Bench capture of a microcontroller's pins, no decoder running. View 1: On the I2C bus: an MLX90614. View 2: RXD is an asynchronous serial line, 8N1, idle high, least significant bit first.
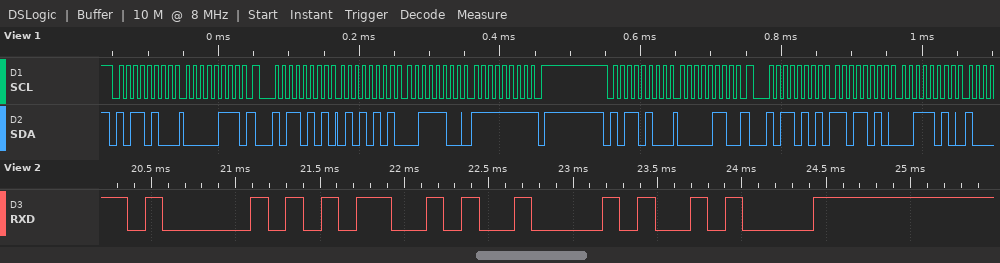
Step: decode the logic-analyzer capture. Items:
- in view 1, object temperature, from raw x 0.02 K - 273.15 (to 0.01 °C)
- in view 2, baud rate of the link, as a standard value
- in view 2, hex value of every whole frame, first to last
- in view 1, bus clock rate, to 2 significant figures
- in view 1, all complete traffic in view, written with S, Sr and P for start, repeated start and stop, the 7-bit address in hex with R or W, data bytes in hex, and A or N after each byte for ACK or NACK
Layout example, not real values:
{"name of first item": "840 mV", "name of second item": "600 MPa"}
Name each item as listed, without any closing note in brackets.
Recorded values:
{"in view 1, object temperature, from raw x 0.02 K - 273.15": "35.75 °C", "in view 2, baud rate of the link, as a standard value": "9600 baud", "in view 2, hex value of every whole frame, first to last": "0x41 0x4D 0x42 0x0A", "in view 1, bus clock rate, to 2 significant figures": "100 kHz", "in view 1, all complete traffic in view, written with S, Sr and P for start, repeated start and stop, the 7-bit address in hex with R or W, data bytes in hex, and A or N after each byte for ACK or NACK": "S 5AW A 07 A Sr 5AR A 55 A 3C A FF N P S 5AW A 06 A Sr 5AR A DA A 3A A"}
